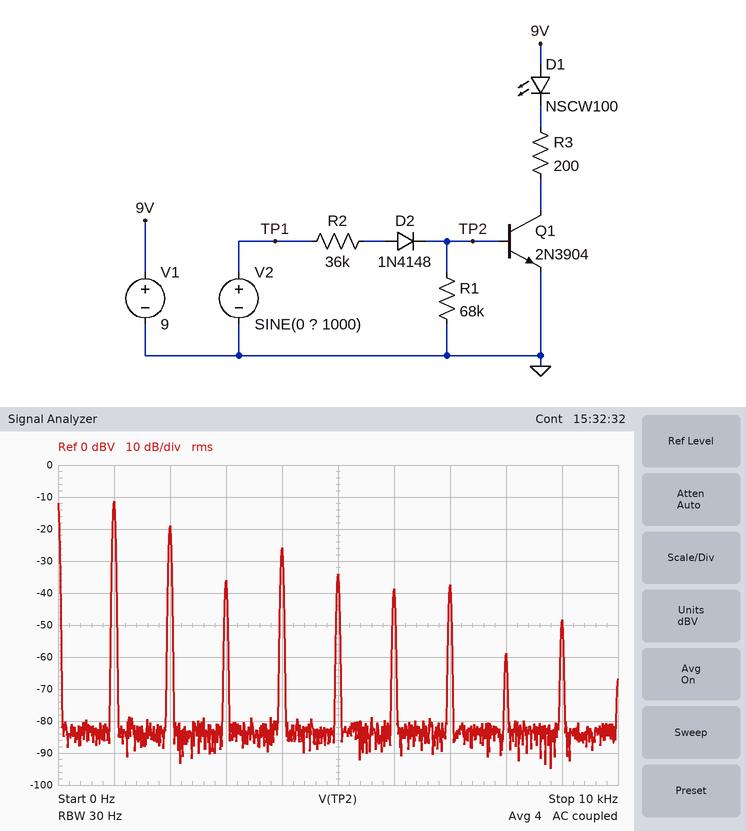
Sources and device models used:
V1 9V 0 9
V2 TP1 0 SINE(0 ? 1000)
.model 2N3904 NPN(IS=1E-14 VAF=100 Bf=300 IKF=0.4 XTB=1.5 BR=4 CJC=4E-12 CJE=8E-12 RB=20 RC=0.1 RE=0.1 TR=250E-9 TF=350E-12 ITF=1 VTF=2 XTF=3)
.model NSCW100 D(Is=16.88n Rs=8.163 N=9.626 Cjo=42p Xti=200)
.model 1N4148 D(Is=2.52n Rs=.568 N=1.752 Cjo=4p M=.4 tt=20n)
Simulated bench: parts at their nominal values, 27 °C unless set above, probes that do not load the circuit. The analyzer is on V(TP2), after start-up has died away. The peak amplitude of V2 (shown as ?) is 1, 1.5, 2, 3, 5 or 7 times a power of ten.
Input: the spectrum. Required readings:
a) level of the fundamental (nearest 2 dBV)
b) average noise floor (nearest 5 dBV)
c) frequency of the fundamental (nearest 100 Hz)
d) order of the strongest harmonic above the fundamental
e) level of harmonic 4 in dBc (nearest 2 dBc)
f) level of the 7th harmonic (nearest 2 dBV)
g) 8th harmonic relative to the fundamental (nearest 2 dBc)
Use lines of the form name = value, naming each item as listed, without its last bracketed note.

level of the fundamental = -12 dBV
average noise floor = -85 dBV
frequency of the fundamental = 1.0 kHz
order of the strongest harmonic above the fundamental = 2
level of harmonic 4 in dBc = -14 dBc
level of the 7th harmonic = -38 dBV
8th harmonic relative to the fundamental = -48 dBc
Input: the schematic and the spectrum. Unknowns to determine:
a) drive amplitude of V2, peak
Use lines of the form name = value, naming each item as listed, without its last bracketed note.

drive amplitude of V2, peak = 2 V
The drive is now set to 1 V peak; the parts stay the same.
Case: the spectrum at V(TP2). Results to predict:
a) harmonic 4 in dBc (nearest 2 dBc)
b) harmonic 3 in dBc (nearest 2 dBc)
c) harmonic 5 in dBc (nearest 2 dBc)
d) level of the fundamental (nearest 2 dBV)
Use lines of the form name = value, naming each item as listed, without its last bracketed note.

harmonic 4 in dBc = -26 dBc
harmonic 3 in dBc = -16 dBc
harmonic 5 in dBc = -24 dBc
level of the fundamental = -18 dBV
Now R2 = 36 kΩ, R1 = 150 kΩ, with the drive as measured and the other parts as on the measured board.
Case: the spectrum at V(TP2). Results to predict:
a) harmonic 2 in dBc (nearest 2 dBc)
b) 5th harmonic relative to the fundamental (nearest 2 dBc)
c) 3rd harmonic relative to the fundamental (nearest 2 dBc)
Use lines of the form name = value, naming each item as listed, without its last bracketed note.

harmonic 2 in dBc = -8 dBc
5th harmonic relative to the fundamental = -28 dBc
3rd harmonic relative to the fundamental = -18 dBc
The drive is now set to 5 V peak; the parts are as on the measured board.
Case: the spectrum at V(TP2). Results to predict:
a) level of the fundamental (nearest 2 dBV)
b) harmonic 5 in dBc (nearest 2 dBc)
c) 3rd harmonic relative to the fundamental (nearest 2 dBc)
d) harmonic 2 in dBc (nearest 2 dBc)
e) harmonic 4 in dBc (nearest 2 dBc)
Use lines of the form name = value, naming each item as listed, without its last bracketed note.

level of the fundamental = -10 dBV
harmonic 5 in dBc = -20 dBc
3rd harmonic relative to the fundamental = -12 dBc
harmonic 2 in dBc = -14 dBc
harmonic 4 in dBc = -16 dBc
